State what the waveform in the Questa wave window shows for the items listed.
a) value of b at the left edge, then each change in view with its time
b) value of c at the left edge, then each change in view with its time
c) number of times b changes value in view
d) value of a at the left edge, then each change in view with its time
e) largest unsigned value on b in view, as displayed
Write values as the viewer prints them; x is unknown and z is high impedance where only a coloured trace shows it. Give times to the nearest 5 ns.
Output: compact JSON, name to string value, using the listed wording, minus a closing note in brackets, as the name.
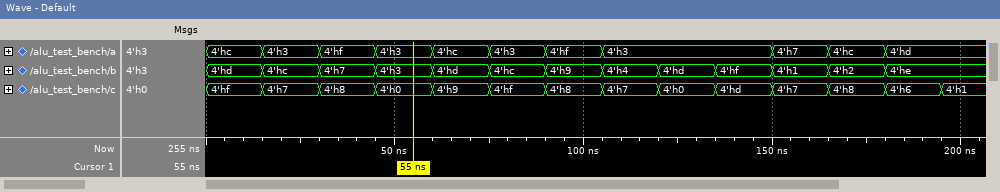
{"value of b at the left edge, then each change in view with its time": "4'hd, 4'hc at 15 ns, 4'h7 at 30 ns, 4'h3 at 45 ns, 4'hd at 60 ns, 4'hc at 75 ns, 4'h9 at 90 ns, 4'h4 at 105 ns, 4'hd at 120 ns, 4'hf at 135 ns, 4'h1 at 150 ns, 4'h2 at 165 ns, 4'he at 180 ns", "value of c at the left edge, then each change in view with its time": "4'hf, 4'h7 at 15 ns, 4'h8 at 30 ns, 4'h0 at 45 ns, 4'h9 at 60 ns, 4'hf at 75 ns, 4'h8 at 90 ns, 4'h7 at 105 ns, 4'h0 at 120 ns, 4'hd at 135 ns, 4'h7 at 150 ns, 4'h8 at 165 ns, 4'h6 at 180 ns, 4'h1 at 195 ns", "number of times b changes value in view": "12", "value of a at the left edge, then each change in view with its time": "4'hc, 4'h3 at 15 ns, 4'hf at 30 ns, 4'h3 at 45 ns, 4'hc at 60 ns, 4'h3 at 75 ns, 4'hf at 90 ns, 4'h3 at 105 ns, 4'h7 at 150 ns, 4'hc at 165 ns, 4'hd at 180 ns", "largest unsigned value on b in view, as displayed": "4'hf"}
